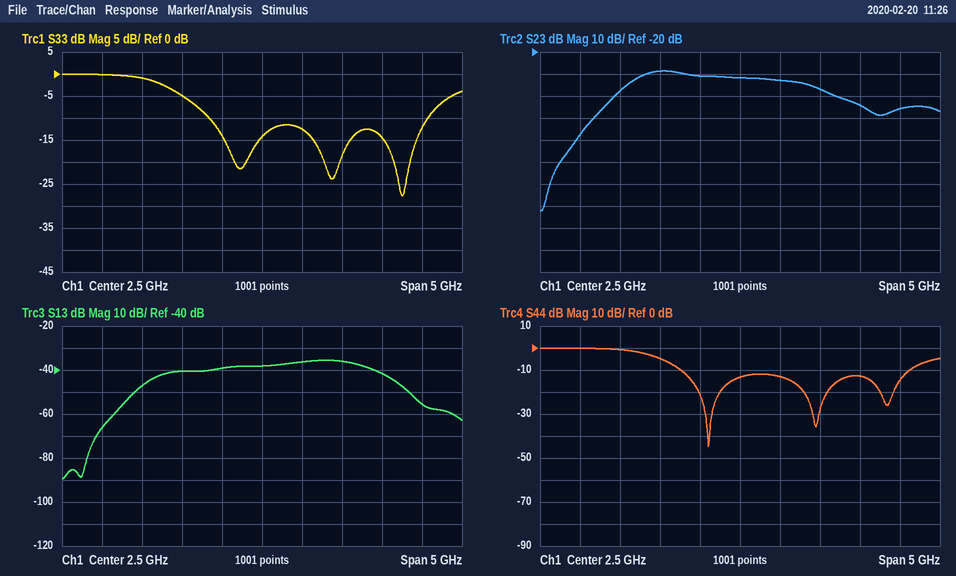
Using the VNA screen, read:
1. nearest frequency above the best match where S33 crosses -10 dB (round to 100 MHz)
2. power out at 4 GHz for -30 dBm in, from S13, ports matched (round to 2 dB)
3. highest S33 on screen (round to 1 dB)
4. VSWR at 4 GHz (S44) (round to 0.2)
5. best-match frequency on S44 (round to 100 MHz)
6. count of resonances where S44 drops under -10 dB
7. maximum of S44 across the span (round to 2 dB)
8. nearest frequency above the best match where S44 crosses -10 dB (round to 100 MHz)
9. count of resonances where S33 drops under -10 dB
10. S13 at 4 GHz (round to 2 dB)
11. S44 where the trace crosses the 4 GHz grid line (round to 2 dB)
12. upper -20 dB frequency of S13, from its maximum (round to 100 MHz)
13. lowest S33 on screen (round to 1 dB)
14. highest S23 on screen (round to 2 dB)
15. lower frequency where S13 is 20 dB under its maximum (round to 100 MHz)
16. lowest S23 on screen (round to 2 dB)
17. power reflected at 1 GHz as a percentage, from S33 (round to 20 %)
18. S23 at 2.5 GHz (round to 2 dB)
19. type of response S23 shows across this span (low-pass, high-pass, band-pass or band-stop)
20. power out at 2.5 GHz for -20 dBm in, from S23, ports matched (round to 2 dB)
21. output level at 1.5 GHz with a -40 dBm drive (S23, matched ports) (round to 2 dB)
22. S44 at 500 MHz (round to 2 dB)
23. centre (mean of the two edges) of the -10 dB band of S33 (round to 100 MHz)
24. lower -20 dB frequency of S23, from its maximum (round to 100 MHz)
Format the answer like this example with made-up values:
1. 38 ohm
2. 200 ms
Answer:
1. 4.6 GHz
2. -72 dBm
3. 0 dB
4. 1.6
5. 2.1 GHz
6. 3
7. 0 dB
8. 4.6 GHz
9. 3
10. -42 dB
11. -12 dB
12. 4.5 GHz
13. -28 dB
14. -28 dB
15. 800 MHz
16. -92 dB
17. 80 %
18. -32 dB
19. band-pass
20. -52 dBm
21. -68 dBm
22. 0 dB
23. 3.2 GHz
24. 700 MHz
